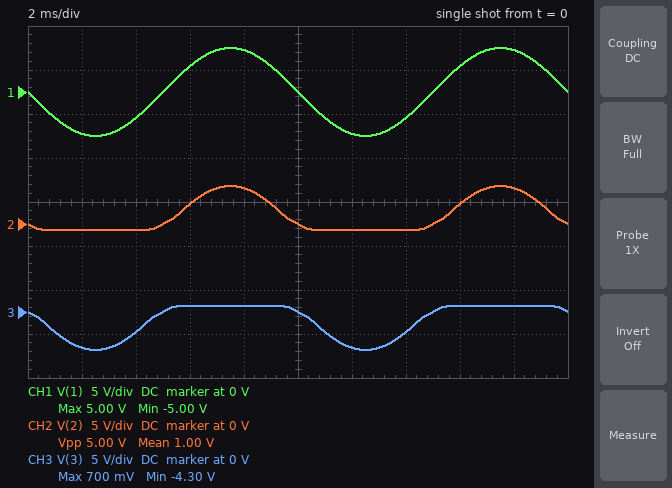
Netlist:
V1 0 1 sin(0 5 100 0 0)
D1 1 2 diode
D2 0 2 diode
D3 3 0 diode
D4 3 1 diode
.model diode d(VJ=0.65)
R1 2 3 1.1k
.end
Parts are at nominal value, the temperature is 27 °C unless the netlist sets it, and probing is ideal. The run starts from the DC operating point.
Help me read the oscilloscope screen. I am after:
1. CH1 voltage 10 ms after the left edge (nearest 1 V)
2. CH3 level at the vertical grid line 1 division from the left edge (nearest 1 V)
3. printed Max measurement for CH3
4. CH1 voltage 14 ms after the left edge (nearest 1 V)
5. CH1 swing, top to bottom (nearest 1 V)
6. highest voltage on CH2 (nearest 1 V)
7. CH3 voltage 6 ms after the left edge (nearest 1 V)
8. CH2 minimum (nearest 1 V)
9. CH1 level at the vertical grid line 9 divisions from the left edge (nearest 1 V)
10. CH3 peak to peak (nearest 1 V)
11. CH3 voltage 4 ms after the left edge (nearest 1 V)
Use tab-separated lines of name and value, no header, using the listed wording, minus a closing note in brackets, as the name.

CH1 voltage 10 ms after the left edge	0 V
CH3 level at the vertical grid line 1 division from the left edge	-4 V
printed Max measurement for CH3	700 mV
CH1 voltage 14 ms after the left edge	-3 V
CH1 swing, top to bottom	10 V
highest voltage on CH2	4 V
CH3 voltage 6 ms after the left edge	1 V
CH2 minimum	-1 V
CH1 level at the vertical grid line 9 divisions from the left edge	5 V
CH3 peak to peak	5 V
CH3 voltage 4 ms after the left edge	-2 V
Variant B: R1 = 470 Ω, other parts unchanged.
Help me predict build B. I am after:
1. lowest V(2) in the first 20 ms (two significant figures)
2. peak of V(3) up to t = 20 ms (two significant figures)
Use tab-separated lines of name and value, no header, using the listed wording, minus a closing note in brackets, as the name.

lowest V(2) in the first 20 ms	-710 mV
peak of V(3) up to t = 20 ms	710 mV
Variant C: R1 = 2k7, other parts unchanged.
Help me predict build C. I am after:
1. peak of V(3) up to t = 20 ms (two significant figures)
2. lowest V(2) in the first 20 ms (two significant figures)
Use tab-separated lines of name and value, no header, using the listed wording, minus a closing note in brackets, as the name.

peak of V(3) up to t = 20 ms	660 mV
lowest V(2) in the first 20 ms	-660 mV
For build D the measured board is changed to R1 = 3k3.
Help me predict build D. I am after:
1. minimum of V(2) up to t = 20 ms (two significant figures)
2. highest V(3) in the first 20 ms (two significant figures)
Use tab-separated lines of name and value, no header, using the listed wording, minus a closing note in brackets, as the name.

minimum of V(2) up to t = 20 ms	-660 mV
highest V(3) in the first 20 ms	660 mV
